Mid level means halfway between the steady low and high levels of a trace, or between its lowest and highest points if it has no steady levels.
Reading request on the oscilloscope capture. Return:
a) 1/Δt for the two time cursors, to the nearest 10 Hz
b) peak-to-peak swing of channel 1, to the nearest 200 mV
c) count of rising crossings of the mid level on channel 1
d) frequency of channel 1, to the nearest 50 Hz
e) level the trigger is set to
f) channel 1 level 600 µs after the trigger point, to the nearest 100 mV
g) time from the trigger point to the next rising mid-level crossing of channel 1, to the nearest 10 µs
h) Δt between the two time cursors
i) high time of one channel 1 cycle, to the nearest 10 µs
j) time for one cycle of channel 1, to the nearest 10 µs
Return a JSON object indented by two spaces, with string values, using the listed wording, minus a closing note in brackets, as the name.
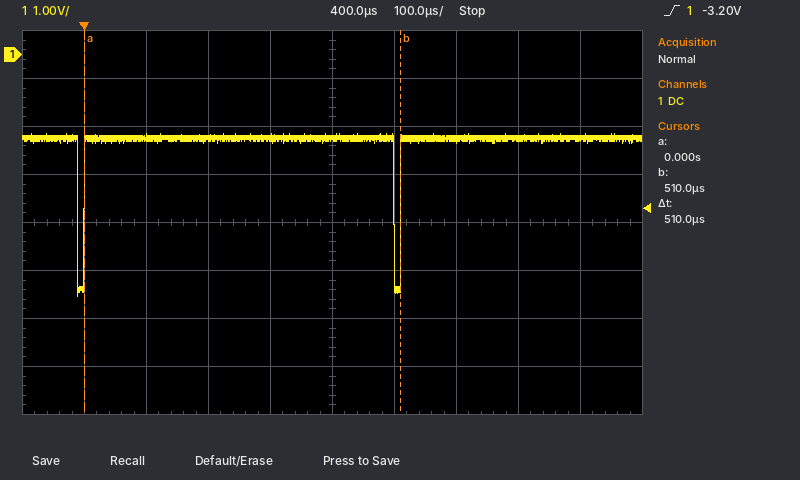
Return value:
{
  "1/Δt for the two time cursors, to the nearest 10 Hz": "1.96 kHz",
  "peak-to-peak swing of channel 1, to the nearest 200 mV": "3.4 V",
  "count of rising crossings of the mid level on channel 1": "2",
  "frequency of channel 1, to the nearest 50 Hz": "1.95 kHz",
  "level the trigger is set to": "-3.20 V",
  "channel 1 level 600 µs after the trigger point, to the nearest 100 mV": "-1.8 V",
  "time from the trigger point to the next rising mid-level crossing of channel 1, to the nearest 10 µs": "510 µs",
  "Δt between the two time cursors": "510 µs",
  "high time of one channel 1 cycle, to the nearest 10 µs": "500 µs",
  "time for one cycle of channel 1, to the nearest 10 µs": "510 µs"
}
